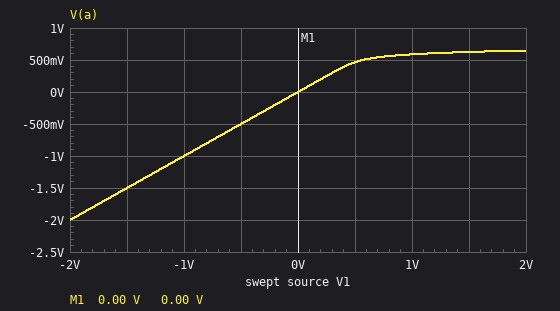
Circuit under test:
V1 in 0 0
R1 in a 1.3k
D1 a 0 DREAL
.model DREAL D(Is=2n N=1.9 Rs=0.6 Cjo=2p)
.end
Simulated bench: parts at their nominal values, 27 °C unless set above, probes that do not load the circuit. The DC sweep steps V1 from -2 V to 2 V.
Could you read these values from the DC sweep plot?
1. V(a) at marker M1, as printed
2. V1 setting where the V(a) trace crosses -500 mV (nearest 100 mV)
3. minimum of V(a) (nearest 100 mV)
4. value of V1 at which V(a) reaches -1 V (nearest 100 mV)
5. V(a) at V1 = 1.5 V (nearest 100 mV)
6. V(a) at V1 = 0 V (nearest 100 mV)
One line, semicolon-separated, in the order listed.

0.00 V; -500 mV; -2.0 V; -1.0 V; 600 mV; 0 V
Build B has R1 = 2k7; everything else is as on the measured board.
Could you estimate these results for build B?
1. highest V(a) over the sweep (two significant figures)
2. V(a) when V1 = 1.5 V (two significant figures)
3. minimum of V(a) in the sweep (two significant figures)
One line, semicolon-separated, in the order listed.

610 mV; 590 mV; -2.0 V
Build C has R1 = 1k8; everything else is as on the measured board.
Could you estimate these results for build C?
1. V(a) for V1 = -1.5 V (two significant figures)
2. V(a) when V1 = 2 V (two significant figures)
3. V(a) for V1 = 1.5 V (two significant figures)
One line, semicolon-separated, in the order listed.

-1.5 V; 630 mV; 610 mV
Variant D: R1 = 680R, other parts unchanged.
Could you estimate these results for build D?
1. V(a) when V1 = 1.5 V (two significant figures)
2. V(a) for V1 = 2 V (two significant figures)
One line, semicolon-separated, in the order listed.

660 mV; 680 mV
